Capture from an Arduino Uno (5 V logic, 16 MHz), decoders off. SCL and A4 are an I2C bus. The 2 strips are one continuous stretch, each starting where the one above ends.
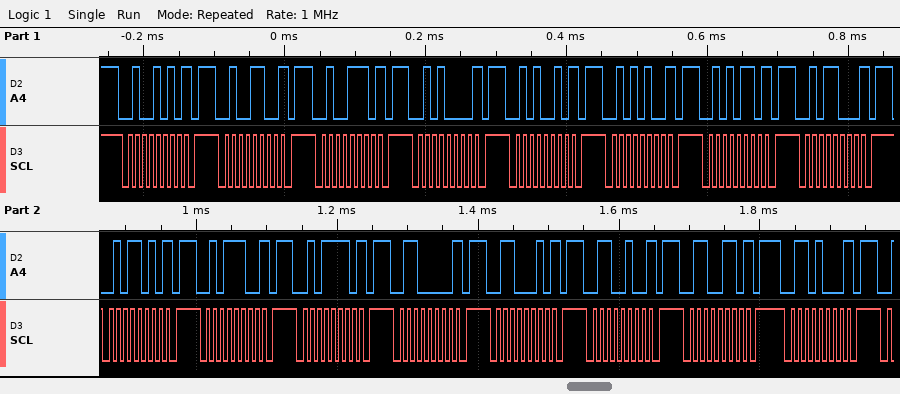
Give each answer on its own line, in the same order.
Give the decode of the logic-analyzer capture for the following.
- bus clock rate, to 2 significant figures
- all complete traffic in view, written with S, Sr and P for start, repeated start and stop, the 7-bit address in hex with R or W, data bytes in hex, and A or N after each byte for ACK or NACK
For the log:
100 kHz
S 25W N P S 26W N P S 27W N P S 28W N P S 29W N P S 2AW N P S 2BW N P S 2CW N P S 2DW N P S 2EW N P S 2FW N P S 30W N P S 31W N P S 32W N P S 33W N P S 34W N P
